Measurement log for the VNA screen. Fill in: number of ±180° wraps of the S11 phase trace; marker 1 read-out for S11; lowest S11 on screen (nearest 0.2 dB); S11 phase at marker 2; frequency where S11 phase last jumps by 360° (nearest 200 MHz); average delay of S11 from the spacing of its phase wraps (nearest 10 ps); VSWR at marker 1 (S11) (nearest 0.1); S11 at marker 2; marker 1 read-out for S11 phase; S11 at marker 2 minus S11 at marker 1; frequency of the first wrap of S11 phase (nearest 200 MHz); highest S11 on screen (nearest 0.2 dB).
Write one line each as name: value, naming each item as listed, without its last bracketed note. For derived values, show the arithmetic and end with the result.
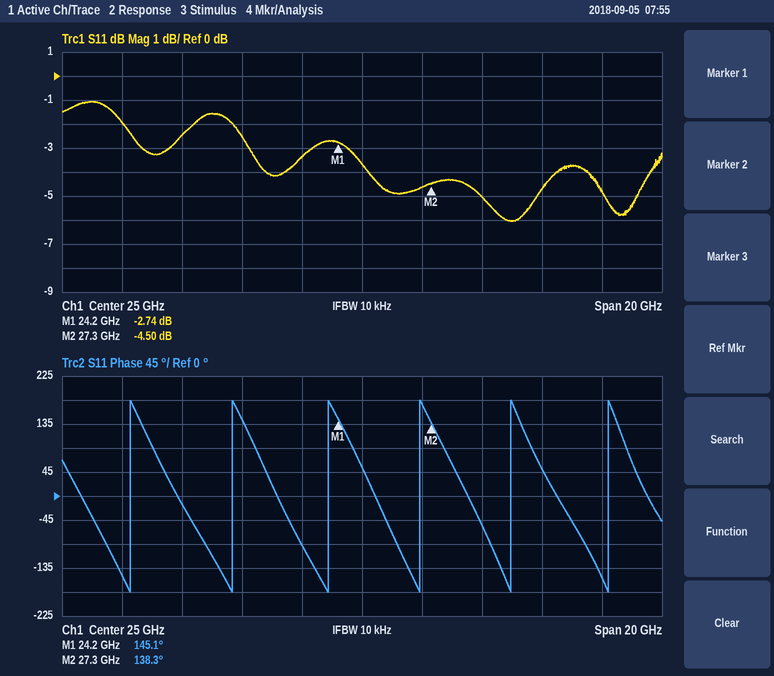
number of ±180° wraps of the S11 phase trace: 6
marker 1 read-out for S11: -2.74 dB
lowest S11 on screen: -6.0 dB
S11 phase at marker 2: 138.3°
frequency where S11 phase last jumps by 360°: 33.2 GHz
average delay of S11 from the spacing of its phase wraps: 5 cycles / (33.2 GHz − 17.2 GHz) ≈ 313 ps, so 310 ps to the nearest 10 ps
VSWR at marker 1 (S11): (1 + 0.7295)/(1 − 0.7295) ≈ 6.4
S11 at marker 2: -4.50 dB
marker 1 read-out for S11 phase: 145.1°
S11 at marker 2 minus S11 at marker 1: -4.5 − (-2.74) = -1.76 dB
frequency of the first wrap of S11 phase: 17.2 GHz
highest S11 on screen: -1.0 dB
